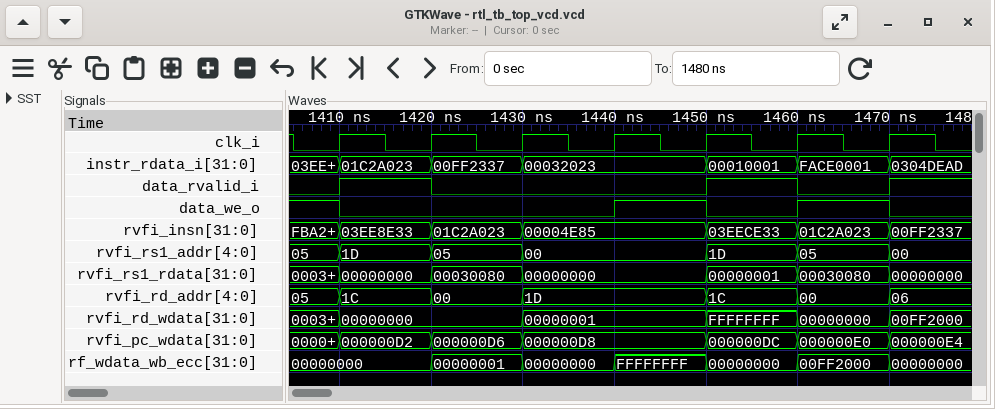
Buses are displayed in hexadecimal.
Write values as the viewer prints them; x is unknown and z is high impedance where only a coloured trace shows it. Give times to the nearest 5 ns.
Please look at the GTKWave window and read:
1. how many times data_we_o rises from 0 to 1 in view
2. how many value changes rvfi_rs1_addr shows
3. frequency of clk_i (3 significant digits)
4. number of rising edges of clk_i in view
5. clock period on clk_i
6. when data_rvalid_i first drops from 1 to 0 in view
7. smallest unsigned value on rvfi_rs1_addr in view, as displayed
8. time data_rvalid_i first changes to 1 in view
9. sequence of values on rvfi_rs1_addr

2
6
100 MHz
7
10 ns
1420 ns
00
1410 ns
05, 1D, 05, 00, 1D, 05, 00
